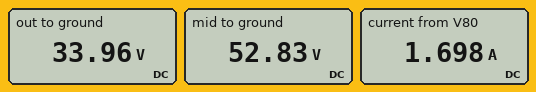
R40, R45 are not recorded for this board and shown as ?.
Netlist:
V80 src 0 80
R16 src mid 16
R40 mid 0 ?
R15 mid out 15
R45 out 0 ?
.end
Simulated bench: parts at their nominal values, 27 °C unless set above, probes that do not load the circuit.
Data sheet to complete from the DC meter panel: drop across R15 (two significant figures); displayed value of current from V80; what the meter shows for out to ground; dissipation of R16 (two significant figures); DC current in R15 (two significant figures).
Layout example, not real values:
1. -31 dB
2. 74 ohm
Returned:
1. 19 V
2. 1.698 A
3. 33.96 V
4. 46 W
5. 1.3 A
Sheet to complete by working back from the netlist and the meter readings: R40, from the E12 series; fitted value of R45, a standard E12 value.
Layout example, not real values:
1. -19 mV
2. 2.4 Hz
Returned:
1. 120 Ω
2. 27 Ω
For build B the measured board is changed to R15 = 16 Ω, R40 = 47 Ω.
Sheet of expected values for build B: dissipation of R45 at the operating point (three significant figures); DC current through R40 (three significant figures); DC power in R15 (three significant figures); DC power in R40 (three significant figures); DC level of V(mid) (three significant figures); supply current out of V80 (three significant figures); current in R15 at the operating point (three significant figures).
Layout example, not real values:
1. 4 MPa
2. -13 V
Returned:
1. 31.9 W
2. 994 mA
3. 18.9 W
4. 46.4 W
5. 46.7 V
6. 2.08 A
7. 1.09 A
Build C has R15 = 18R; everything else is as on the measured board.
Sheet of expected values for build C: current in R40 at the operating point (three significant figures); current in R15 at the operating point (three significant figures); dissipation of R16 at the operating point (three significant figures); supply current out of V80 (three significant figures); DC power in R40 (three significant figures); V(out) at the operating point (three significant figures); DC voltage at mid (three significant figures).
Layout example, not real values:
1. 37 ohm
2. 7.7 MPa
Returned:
1. 448 mA
2. 1.19 A
3. 43.1 W
4. 1.64 A
5. 24.1 W
6. 32.2 V
7. 53.7 V
